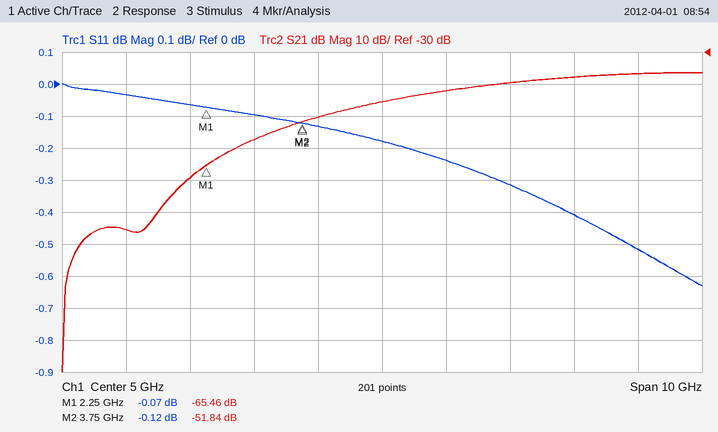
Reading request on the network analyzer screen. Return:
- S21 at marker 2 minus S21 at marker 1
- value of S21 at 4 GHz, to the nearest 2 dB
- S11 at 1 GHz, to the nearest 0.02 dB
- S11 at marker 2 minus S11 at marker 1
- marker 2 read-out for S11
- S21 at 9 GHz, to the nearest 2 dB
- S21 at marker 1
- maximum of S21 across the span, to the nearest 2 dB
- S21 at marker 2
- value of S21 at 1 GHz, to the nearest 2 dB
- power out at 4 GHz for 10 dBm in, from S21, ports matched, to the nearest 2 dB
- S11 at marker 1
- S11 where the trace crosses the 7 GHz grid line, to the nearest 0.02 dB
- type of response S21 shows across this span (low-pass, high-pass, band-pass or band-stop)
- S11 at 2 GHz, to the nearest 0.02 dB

13.62 dB
-50 dB
-0.04 dB
-0.05 dB
-0.12 dB
-36 dB
-65.46 dB
-36 dB
-51.84 dB
-86 dB
-40 dBm
-0.07 dB
-0.32 dB
high-pass
-0.06 dB
